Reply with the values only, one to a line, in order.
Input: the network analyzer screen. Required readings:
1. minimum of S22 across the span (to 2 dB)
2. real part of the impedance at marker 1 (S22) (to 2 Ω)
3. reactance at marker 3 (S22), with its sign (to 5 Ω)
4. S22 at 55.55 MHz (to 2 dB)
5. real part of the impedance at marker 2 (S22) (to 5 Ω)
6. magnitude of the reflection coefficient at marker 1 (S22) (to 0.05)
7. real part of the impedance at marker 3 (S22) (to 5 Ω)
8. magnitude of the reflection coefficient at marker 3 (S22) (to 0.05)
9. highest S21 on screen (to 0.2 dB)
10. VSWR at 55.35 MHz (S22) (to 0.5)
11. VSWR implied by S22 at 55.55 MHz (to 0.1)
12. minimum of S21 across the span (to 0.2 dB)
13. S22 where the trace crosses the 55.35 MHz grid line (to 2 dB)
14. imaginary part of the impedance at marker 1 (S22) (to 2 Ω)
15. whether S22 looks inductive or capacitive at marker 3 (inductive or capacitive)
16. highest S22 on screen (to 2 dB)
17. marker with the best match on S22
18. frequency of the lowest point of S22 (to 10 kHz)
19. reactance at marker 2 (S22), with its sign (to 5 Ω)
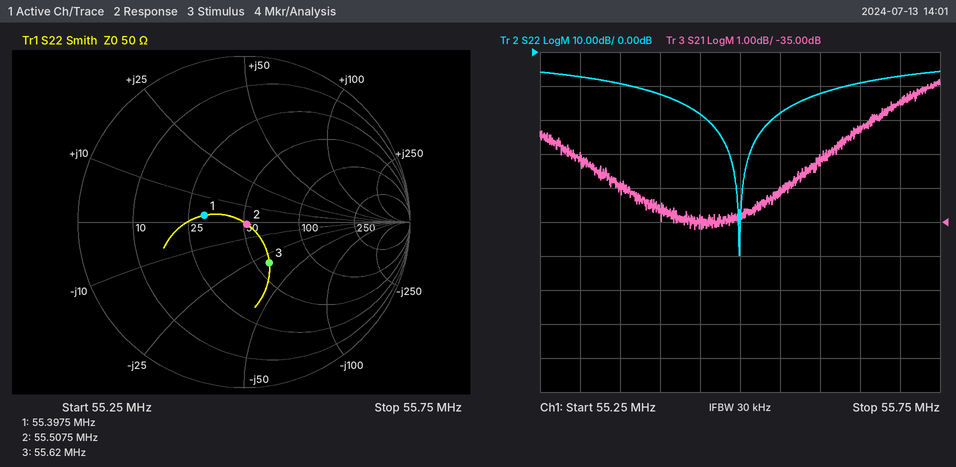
-60 dB
30 Ω
-30 Ω
-18 dB
50 Ω
0.25
60 Ω
0.30
-30.8 dB
2.0
1.3
-35.2 dB
-10 dB
+2 Ω
capacitive
-6 dB
marker 2
55.50 MHz
0 Ω
